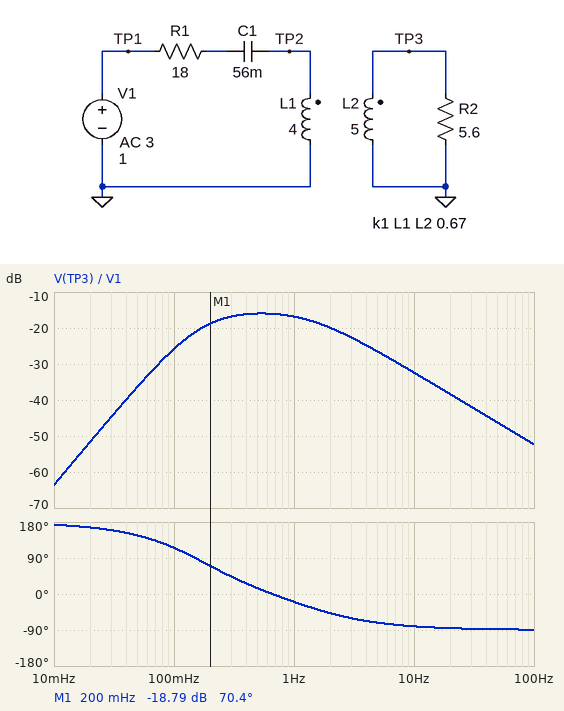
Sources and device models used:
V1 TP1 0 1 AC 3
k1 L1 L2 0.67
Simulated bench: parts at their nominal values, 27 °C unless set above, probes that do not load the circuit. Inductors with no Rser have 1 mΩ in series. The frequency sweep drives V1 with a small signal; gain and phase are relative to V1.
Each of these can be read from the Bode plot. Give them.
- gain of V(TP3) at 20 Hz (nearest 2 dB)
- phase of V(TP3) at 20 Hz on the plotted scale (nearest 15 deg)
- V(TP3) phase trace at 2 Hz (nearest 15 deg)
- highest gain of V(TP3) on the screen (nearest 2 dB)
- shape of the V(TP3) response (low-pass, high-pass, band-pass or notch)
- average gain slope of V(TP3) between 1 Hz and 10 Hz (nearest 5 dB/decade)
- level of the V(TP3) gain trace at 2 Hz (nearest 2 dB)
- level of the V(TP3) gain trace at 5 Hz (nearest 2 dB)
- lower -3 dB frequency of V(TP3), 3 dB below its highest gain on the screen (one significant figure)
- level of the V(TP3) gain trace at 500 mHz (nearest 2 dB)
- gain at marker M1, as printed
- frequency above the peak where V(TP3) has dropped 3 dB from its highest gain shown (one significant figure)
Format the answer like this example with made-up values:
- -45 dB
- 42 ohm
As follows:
- -38 dB
- -90 deg
- -45 deg
- -16 dB
- band-pass
- -15 dB/decade
- -20 dB
- -26 dB
- 200 mHz
- -16 dB
- -18.79 dB
- 2 Hz
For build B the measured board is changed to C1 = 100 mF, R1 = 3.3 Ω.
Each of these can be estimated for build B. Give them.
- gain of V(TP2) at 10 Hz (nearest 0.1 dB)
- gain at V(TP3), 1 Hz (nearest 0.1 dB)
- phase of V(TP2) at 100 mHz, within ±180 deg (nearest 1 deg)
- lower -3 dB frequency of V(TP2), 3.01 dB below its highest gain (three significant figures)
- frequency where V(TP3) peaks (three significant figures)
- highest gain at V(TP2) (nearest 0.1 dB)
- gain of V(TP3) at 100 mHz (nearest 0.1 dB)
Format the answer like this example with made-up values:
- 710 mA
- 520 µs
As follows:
- 0 dB
- -12.3 dB
- 152 deg
- 234 mHz
- 317 mHz
- 1.5 dB
- -18.7 dB
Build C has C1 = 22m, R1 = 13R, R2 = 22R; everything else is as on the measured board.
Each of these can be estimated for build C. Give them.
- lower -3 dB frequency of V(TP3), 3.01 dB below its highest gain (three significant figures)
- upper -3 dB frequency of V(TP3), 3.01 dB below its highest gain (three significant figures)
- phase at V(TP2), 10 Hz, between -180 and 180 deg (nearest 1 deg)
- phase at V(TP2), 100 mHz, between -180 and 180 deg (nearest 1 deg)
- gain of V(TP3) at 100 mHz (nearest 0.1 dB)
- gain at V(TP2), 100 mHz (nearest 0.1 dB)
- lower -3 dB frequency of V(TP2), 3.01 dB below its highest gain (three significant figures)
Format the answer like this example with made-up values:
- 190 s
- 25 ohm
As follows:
- 407 mHz
- 1.93 Hz
- 5 deg
- 166 deg
- -31.6 dB
- -29.1 dB
- 522 mHz
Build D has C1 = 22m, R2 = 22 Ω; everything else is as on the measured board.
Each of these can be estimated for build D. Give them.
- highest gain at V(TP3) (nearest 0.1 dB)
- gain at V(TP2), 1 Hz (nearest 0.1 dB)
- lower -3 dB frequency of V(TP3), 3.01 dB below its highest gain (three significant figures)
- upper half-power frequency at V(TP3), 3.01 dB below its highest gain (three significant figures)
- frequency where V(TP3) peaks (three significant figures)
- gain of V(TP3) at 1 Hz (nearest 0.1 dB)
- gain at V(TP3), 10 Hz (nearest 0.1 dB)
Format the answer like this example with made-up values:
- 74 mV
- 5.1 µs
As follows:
- -7.4 dB
- -2.9 dB
- 405 mHz
- 2.48 Hz
- 856 mHz
- -7.5 dB
- -20.6 dB
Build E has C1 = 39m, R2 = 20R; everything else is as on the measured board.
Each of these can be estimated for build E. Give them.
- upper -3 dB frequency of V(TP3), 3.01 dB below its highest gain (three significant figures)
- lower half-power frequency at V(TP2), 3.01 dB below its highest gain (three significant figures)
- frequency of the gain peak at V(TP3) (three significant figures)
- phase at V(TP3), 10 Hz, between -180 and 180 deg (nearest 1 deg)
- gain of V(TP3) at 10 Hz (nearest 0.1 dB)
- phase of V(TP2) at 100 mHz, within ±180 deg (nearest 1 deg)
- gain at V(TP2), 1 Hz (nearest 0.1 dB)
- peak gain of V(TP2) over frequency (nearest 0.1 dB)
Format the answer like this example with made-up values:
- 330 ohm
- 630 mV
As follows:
- 2.50 Hz
- 1.17 Hz
- 816 mHz
- -76 deg
- -21.4 dB
- 151 deg
- -3.4 dB
- 0 dB
